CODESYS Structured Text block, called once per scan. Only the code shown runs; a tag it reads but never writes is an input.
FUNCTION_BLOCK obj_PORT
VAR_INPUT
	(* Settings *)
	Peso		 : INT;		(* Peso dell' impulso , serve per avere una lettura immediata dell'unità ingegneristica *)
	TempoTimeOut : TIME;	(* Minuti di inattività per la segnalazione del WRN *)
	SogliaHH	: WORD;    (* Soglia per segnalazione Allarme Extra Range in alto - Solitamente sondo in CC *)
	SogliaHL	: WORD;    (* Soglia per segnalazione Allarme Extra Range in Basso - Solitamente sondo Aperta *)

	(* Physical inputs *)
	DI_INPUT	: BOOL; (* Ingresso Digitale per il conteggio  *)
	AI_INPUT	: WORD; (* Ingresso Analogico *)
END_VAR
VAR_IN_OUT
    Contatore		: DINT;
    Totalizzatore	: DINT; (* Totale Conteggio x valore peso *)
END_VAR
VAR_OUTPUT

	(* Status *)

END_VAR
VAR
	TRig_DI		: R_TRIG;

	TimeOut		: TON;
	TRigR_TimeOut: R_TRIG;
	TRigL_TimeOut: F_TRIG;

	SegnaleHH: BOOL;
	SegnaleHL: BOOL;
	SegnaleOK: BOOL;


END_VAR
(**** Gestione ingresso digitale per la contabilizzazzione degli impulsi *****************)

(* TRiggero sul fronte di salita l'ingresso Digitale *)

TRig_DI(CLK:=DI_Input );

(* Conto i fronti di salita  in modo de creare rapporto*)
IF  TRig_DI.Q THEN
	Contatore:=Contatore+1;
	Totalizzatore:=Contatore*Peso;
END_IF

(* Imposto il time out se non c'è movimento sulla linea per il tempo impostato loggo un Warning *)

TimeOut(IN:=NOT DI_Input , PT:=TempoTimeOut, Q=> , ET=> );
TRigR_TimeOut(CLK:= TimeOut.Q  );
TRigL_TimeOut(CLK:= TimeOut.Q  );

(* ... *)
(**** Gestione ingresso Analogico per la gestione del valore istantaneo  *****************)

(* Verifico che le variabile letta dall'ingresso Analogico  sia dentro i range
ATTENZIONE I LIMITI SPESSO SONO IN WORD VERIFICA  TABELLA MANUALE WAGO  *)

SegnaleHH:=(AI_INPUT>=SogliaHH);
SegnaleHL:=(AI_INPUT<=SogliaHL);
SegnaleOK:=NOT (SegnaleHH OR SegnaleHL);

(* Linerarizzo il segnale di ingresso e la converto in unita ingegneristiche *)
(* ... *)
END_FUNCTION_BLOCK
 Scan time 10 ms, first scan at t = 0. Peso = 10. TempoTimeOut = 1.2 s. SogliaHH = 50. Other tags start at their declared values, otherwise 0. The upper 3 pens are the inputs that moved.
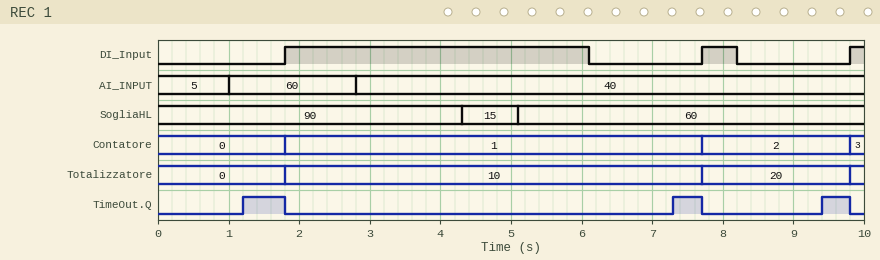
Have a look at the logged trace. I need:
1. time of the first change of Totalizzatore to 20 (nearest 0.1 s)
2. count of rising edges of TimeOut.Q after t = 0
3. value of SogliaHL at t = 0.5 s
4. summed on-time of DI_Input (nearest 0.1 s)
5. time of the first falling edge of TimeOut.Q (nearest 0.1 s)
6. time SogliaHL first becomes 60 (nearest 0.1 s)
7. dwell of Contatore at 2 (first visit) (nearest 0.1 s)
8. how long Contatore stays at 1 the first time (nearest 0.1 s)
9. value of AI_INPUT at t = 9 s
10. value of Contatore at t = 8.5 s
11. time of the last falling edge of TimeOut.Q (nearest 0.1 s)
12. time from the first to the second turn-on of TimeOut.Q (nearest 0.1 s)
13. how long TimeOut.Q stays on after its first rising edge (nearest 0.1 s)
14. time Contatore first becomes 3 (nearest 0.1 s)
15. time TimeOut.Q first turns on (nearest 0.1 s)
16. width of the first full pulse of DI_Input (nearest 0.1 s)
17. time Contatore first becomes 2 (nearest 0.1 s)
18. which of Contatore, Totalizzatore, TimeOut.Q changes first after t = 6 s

7.7 s
3
90
5.0 s
1.8 s
5.1 s
2.1 s
5.9 s
40
2
9.8 s
6.1 s
0.6 s
9.8 s
1.2 s
4.3 s
7.7 s
TimeOut.Q
